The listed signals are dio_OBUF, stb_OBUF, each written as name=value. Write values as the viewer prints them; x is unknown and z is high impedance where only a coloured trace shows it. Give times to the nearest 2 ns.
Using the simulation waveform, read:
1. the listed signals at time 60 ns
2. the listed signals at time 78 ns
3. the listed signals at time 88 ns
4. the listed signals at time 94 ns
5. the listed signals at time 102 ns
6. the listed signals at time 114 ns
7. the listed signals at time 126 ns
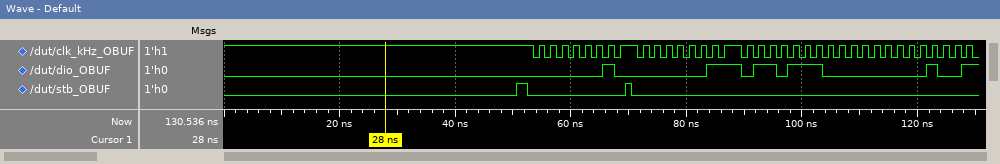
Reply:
dio_OBUF=0, stb_OBUF=0
dio_OBUF=0, stb_OBUF=0
dio_OBUF=1, stb_OBUF=0
dio_OBUF=1, stb_OBUF=0
dio_OBUF=1, stb_OBUF=0
dio_OBUF=0, stb_OBUF=0
dio_OBUF=0, stb_OBUF=0
